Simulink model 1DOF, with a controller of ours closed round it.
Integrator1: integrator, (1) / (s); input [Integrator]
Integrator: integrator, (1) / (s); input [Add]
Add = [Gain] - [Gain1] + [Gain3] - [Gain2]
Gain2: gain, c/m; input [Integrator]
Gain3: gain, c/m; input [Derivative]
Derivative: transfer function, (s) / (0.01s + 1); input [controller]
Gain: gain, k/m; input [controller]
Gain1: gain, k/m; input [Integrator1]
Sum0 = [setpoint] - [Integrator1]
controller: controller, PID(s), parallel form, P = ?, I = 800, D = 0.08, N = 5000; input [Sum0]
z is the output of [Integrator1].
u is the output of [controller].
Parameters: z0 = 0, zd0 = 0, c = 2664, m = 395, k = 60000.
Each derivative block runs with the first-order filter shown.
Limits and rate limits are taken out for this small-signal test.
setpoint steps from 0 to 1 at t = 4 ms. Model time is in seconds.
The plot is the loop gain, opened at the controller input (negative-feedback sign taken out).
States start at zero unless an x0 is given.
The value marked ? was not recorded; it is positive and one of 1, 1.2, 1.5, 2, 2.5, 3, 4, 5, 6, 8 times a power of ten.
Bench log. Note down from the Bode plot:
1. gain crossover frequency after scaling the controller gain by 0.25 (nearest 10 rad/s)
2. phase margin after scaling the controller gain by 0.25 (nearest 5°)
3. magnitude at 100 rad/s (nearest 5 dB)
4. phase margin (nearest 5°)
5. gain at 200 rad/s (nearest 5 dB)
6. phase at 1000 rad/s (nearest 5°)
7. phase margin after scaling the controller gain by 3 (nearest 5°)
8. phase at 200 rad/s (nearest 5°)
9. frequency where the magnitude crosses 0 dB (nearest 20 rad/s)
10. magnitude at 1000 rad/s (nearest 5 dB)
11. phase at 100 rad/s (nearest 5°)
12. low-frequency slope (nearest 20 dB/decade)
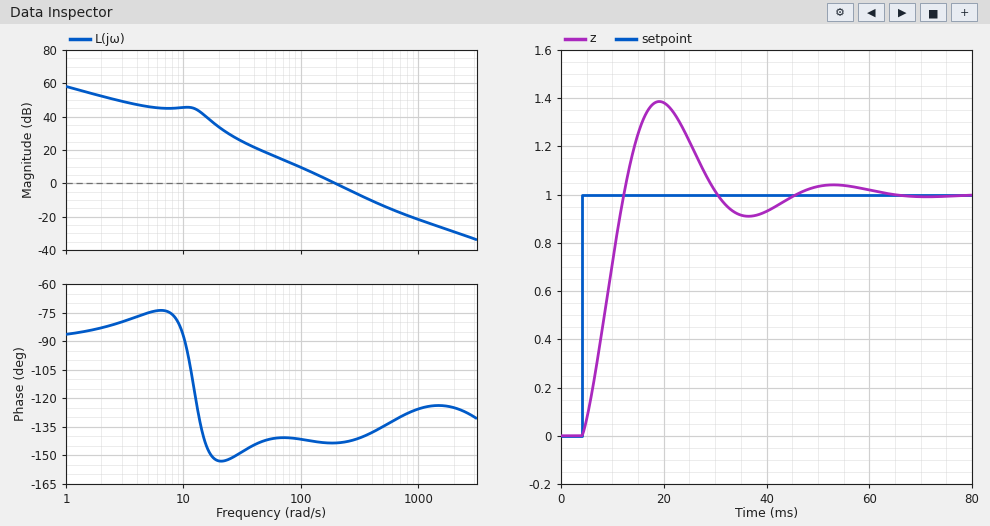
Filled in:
80 rad/s
40°
10 dB
35°
0 dB
-125°
40°
-145°
200 rad/s
-20 dB
-140°
-20 dB/decade
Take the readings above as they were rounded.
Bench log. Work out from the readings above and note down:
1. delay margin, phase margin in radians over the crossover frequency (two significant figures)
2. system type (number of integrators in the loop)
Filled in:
0.0031 s
1
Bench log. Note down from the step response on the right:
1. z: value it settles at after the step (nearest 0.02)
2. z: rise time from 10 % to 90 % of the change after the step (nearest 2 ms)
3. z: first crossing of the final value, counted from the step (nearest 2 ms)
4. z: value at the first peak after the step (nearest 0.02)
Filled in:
1.00
6 ms
8 ms
1.38
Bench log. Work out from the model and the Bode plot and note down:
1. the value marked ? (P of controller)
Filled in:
50
